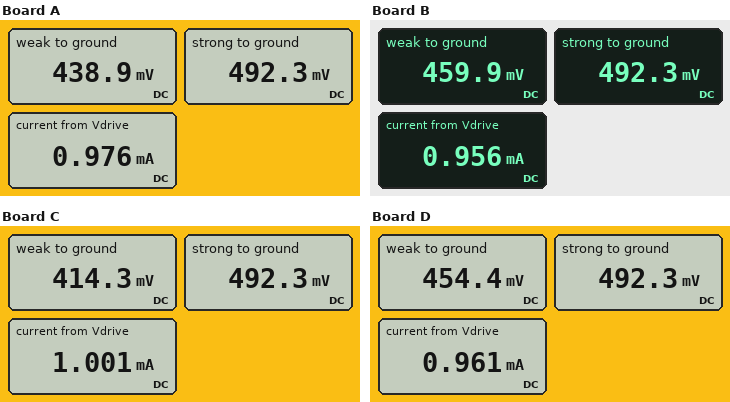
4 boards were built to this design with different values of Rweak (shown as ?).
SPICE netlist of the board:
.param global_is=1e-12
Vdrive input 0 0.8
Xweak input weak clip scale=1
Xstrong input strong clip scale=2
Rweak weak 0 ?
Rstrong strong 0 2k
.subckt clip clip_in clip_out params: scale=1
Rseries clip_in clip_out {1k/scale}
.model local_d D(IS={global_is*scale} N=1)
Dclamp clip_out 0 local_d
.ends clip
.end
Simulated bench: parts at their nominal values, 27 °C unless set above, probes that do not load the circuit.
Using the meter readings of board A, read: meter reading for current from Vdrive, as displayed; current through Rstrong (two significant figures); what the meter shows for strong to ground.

0.976 mA
250 µA
492.3 mV
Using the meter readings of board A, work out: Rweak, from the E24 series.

1.3 kΩ
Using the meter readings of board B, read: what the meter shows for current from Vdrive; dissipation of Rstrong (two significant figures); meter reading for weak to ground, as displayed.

0.956 mA
120 µW
459.9 mV
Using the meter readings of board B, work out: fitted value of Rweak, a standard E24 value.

1.6 kΩ
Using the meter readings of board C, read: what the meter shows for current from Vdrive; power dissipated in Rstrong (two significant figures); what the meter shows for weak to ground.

1.001 mA
120 µW
414.3 mV
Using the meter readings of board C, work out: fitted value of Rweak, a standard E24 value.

1.1 kΩ
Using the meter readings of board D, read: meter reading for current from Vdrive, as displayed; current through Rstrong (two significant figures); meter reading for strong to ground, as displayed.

0.961 mA
250 µA
492.3 mV
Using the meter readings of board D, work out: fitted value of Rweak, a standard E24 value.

1.5 kΩ
